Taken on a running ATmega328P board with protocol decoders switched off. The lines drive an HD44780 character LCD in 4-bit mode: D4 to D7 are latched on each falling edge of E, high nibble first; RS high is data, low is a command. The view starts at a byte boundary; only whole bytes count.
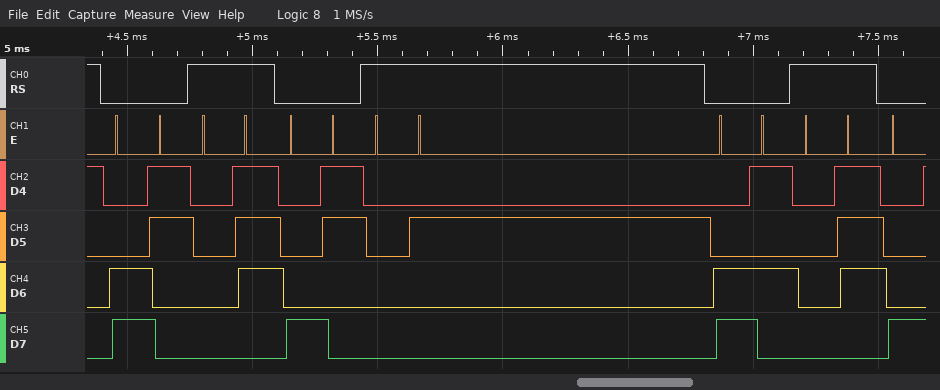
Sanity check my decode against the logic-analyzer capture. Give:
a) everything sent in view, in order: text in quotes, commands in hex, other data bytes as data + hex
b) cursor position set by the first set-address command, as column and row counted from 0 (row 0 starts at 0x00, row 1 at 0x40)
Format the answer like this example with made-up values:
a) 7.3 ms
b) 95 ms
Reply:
a) 0xC3 data 07 0x83 data 02 0xC5 data 07
b) column 3, row 1
